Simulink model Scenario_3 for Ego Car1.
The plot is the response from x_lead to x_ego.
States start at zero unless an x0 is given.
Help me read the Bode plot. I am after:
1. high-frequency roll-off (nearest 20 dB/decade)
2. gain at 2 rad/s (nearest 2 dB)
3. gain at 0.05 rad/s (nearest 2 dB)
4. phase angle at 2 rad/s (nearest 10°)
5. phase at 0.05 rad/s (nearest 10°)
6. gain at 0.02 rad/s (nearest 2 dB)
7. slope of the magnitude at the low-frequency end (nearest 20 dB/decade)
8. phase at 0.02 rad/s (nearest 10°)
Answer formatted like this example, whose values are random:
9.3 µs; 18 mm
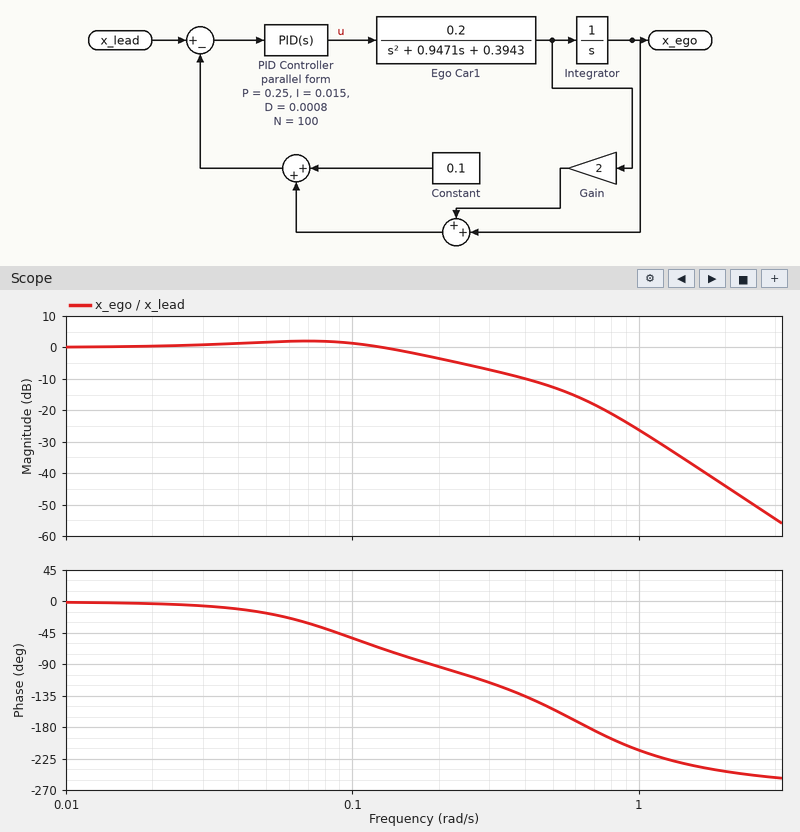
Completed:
-60 dB/decade; -44 dB; 2 dB; -240°; -20°; 0 dB; 0 dB/decade; 0°
